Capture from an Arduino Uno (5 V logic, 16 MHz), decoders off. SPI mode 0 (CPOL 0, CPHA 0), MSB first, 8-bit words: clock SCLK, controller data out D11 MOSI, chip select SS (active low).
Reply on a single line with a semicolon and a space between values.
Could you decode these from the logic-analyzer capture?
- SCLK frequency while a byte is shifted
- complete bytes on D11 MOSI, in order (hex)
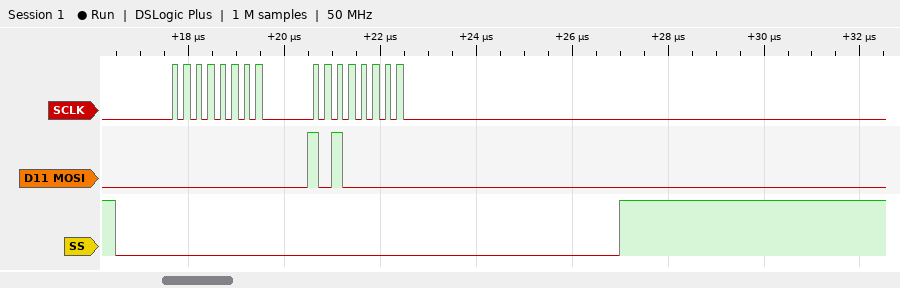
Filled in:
4 MHz; 00 A0
